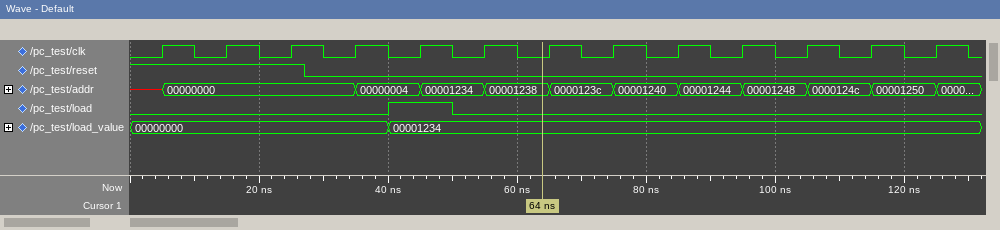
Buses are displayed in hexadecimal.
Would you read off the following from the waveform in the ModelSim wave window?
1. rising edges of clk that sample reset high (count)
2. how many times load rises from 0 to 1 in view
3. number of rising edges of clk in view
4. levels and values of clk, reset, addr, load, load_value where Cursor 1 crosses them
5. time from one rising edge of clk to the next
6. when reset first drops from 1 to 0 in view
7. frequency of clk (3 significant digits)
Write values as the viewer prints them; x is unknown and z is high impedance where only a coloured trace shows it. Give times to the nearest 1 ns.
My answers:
3
1
13
clk=0, reset=0, addr=00001238, load=0, load_value=00001234
10 ns
27 ns
100 MHz
